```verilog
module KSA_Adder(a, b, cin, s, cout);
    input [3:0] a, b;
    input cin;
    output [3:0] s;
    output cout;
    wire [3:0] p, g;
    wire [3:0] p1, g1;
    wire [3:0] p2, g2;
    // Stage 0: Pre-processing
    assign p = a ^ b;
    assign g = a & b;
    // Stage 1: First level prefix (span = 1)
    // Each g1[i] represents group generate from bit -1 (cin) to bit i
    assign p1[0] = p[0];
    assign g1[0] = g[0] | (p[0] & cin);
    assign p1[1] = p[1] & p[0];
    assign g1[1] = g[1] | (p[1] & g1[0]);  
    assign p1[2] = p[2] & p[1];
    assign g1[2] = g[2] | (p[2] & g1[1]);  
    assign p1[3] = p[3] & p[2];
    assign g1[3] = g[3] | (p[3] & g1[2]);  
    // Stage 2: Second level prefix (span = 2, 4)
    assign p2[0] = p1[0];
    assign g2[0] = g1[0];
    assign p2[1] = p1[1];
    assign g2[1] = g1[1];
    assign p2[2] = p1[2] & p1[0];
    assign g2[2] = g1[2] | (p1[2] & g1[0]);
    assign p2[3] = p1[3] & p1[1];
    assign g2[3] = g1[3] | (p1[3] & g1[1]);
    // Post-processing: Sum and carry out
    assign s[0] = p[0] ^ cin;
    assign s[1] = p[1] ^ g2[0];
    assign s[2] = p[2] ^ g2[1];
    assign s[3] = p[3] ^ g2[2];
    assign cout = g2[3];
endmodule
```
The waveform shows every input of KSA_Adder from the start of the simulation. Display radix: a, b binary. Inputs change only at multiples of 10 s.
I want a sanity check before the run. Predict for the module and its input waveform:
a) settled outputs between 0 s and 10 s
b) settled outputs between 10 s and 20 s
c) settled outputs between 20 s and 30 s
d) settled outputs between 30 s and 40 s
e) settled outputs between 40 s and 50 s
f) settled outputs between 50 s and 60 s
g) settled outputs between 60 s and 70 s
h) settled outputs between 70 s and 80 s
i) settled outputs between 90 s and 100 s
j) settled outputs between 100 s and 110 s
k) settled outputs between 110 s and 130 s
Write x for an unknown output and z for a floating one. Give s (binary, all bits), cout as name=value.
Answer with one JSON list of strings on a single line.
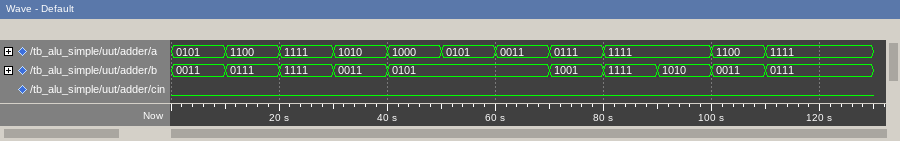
["s=1000, cout=0", "s=0011, cout=1", "s=1110, cout=1", "s=1101, cout=0", "s=1101, cout=0", "s=1010, cout=0", "s=1000, cout=0", "s=0000, cout=1", "s=1001, cout=1", "s=1111, cout=0", "s=0110, cout=1"]
